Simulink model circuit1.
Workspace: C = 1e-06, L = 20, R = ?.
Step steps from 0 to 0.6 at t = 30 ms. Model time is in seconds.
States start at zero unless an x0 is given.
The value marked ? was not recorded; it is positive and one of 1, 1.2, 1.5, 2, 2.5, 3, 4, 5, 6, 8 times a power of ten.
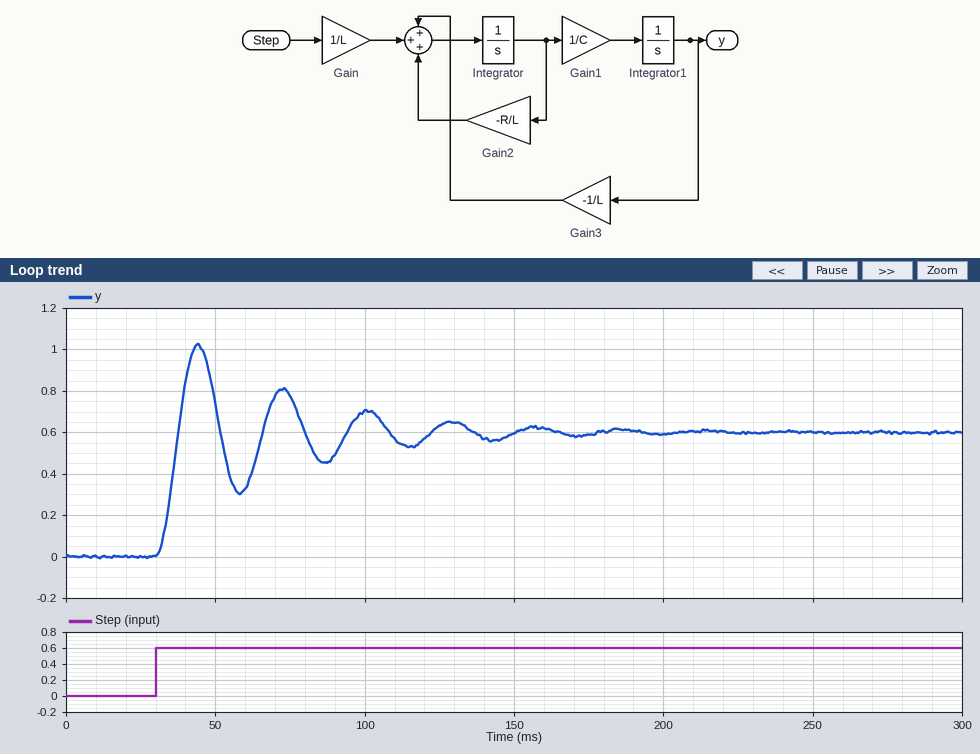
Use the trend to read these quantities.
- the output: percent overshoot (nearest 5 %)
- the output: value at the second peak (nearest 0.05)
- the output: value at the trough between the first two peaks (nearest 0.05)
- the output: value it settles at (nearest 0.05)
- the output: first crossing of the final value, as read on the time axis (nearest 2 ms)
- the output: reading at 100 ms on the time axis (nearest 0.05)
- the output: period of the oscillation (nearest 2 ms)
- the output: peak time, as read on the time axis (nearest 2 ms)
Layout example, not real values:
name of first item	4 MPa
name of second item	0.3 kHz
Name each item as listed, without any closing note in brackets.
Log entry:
the output: percent overshoot	70 %
the output: value at the second peak	0.80
the output: value at the trough between the first two peaks	0.30
the output: value it settles at	0.60
the output: first crossing of the final value, as read on the time axis	38 ms
the output: reading at 100 ms on the time axis	0.70
the output: period of the oscillation	28 ms
the output: peak time, as read on the time axis	44 ms
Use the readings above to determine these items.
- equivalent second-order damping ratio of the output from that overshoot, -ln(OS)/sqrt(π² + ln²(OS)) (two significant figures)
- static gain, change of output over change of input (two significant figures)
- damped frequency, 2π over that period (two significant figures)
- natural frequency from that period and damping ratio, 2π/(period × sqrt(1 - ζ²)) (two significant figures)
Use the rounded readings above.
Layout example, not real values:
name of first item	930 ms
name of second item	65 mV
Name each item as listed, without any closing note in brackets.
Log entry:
equivalent second-order damping ratio of the output from that overshoot, -ln(OS)/sqrt(π² + ln²(OS))	0.11
static gain, change of output over change of input	1.0
damped frequency, 2π over that period	0.22 rad/ms
natural frequency from that period and damping ratio, 2π/(period × sqrt(1 - ζ²))	0.23 rad/ms
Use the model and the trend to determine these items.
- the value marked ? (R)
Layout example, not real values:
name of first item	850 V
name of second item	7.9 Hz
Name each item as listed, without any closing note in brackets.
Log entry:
the value marked ?	1000
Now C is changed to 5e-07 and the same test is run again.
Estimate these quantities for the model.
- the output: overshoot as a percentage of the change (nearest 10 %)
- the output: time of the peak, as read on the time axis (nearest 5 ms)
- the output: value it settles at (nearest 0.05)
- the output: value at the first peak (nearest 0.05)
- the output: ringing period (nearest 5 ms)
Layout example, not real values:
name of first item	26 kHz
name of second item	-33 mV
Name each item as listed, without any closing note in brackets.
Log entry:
the output: overshoot as a percentage of the change	80 %
the output: time of the peak, as read on the time axis	40 ms
the output: value it settles at	0.60
the output: value at the first peak	1.05
the output: ringing period	20 ms
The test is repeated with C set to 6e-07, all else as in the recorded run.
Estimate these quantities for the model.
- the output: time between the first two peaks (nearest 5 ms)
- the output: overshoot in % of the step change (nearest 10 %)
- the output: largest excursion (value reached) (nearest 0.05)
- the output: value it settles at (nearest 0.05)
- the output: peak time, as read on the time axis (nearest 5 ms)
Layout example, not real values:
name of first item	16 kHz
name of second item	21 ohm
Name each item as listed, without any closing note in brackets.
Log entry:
the output: time between the first two peaks	20 ms
the output: overshoot in % of the step change	80 %
the output: largest excursion (value reached)	1.05
the output: value it settles at	0.60
the output: peak time, as read on the time axis	40 ms
